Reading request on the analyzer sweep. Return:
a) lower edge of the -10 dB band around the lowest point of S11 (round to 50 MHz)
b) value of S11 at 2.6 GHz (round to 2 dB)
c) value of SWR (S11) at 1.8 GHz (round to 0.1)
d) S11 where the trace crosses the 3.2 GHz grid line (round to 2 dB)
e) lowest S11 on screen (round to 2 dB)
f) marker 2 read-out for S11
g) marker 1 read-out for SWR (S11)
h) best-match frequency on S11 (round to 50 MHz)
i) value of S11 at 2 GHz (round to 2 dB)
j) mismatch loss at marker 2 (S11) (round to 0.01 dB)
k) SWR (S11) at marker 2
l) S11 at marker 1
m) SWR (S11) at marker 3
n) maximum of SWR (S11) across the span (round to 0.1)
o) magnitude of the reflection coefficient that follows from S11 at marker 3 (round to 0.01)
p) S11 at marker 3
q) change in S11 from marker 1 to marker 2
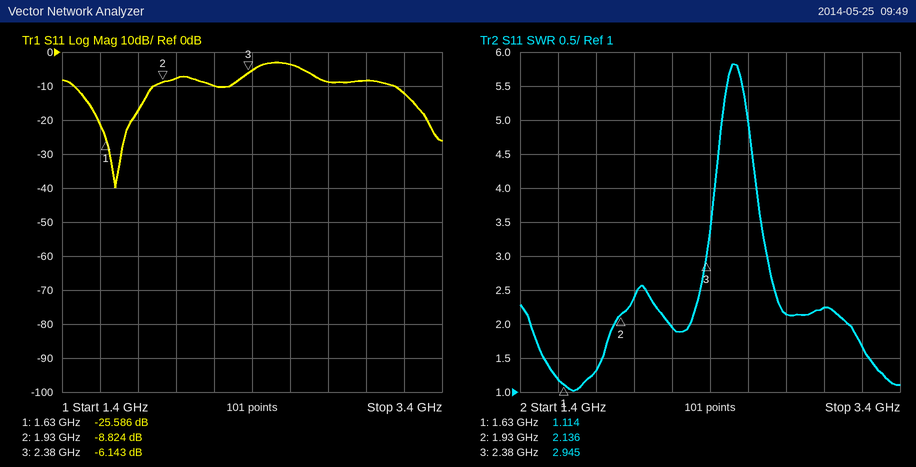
1.45 GHz
-4 dB
1.3
-12 dB
-40 dB
-8.824 dB
1.114
1.70 GHz
-8 dB
0.61 dB
2.136
-25.586 dB
2.945
5.8
0.49
-6.143 dB
16.762 dB
